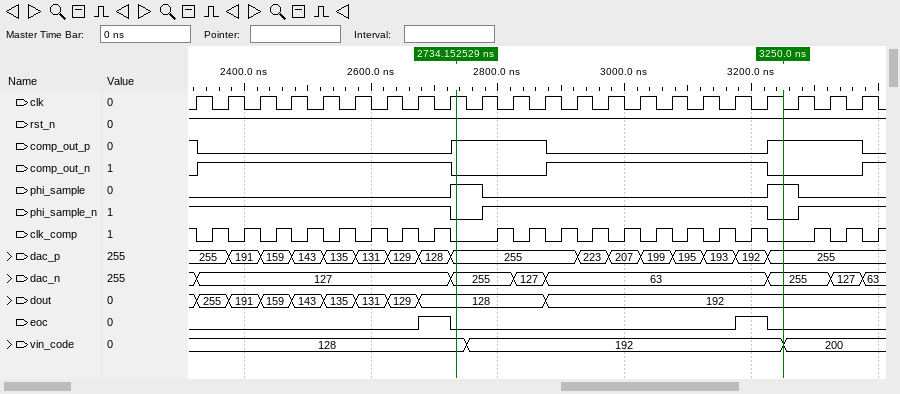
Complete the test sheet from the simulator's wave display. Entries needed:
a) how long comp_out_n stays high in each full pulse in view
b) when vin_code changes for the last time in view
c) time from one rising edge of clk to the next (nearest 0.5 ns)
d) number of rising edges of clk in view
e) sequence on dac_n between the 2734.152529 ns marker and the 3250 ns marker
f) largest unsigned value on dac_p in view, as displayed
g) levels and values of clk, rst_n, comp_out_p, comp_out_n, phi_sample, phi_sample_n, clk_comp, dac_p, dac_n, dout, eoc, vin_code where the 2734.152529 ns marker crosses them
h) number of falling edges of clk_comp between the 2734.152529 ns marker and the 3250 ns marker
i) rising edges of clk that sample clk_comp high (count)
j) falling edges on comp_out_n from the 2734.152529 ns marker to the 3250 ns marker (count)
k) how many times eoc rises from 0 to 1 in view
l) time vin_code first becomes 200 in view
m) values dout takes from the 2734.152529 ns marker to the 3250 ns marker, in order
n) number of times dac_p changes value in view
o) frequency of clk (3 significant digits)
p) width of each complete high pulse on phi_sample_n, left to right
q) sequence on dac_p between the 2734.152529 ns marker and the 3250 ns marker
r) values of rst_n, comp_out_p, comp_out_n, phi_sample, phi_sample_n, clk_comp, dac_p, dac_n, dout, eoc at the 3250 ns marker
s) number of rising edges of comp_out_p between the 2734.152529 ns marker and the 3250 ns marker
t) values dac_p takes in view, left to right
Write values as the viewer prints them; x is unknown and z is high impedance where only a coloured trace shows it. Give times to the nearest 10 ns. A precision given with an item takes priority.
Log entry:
400 ns, 350 ns
3250 ns
50 ns
22
255, 127, 63, 255
255
clk=1, rst_n=1, comp_out_p=1, comp_out_n=0, phi_sample=1, phi_sample_n=0, clk_comp=0, dac_p=255, dac_n=255, dout=128, eoc=0, vin_code=128
9
20
1
2
3250 ns
128, 192
15
20.0 MHz
450 ns
255, 223, 207, 199, 195, 193, 192, 255
rst_n=1, comp_out_p=1, comp_out_n=0, phi_sample=1, phi_sample_n=0, clk_comp=0, dac_p=255, dac_n=255, dout=192, eoc=0
1
255, 191, 159, 143, 135, 131, 129, 128, 255, 223, 207, 199, 195, 193, 192, 255
